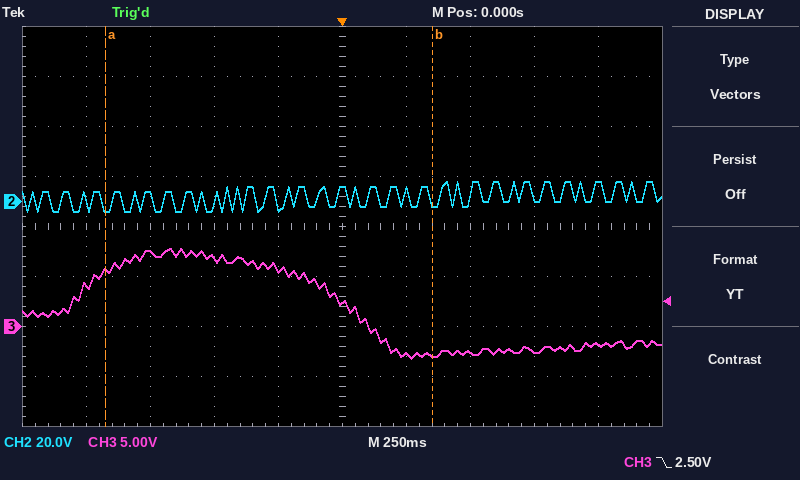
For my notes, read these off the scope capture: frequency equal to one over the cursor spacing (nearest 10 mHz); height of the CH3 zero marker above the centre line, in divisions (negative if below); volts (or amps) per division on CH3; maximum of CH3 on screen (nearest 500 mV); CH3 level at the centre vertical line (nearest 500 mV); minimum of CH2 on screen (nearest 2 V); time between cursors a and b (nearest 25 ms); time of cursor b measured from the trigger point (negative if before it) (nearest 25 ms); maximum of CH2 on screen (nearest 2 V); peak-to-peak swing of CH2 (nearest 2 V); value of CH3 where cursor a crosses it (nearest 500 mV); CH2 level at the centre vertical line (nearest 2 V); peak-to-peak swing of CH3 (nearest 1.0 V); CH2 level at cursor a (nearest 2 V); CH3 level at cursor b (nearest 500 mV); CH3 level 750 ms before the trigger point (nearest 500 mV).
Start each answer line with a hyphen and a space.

- 780 mHz
- -2.0 div
- 5 V
- 8.0 V
- 2.5 V
- -4 V
- 1.275 s
- +350 ms
- 8 V
- 12 V
- 5.5 V
- 6 V
- 11.0 V
- -2 V
- -3.0 V
- 7.5 V
